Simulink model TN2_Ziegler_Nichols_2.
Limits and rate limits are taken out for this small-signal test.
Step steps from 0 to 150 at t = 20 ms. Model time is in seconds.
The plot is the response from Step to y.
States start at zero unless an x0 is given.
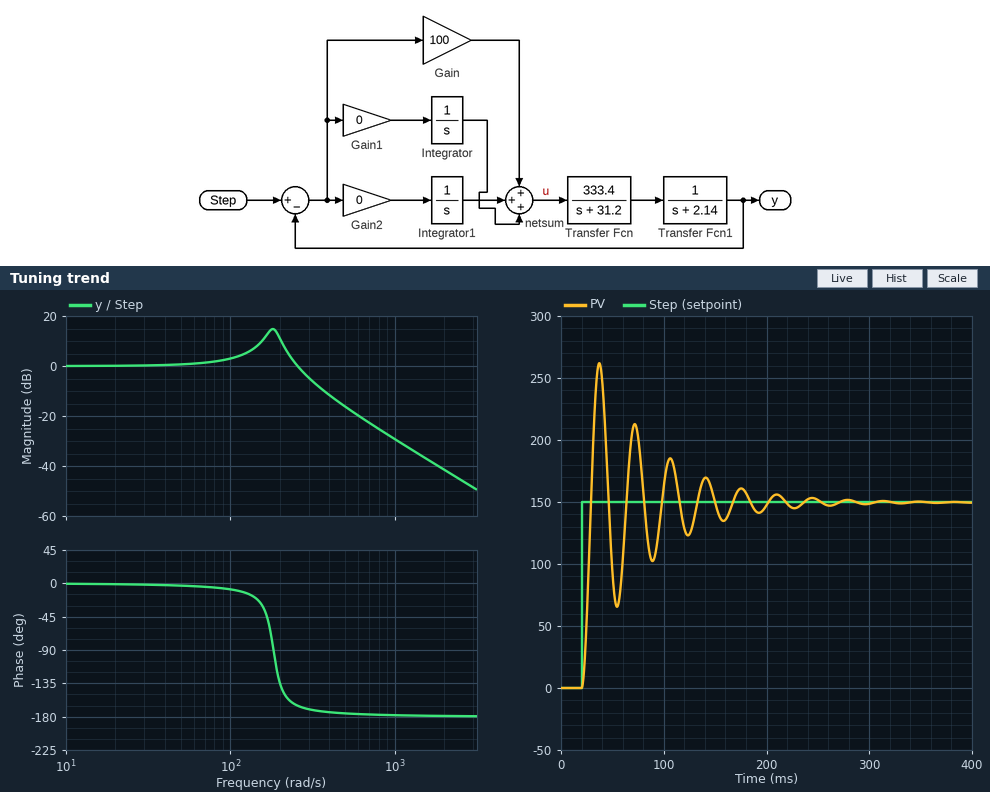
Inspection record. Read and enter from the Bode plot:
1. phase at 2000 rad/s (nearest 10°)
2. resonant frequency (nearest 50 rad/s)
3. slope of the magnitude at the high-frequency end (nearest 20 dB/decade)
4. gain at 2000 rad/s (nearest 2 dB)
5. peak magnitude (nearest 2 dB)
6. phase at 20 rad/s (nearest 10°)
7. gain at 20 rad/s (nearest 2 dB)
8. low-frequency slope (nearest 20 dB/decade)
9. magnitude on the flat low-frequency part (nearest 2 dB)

-180°
200 rad/s
-40 dB/decade
-42 dB
14 dB
0°
0 dB
0 dB/decade
0 dB
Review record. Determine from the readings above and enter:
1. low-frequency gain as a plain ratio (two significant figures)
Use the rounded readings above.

1.0
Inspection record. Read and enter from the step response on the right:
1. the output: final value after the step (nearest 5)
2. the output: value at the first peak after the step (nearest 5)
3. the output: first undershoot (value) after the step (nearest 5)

150
260
65
